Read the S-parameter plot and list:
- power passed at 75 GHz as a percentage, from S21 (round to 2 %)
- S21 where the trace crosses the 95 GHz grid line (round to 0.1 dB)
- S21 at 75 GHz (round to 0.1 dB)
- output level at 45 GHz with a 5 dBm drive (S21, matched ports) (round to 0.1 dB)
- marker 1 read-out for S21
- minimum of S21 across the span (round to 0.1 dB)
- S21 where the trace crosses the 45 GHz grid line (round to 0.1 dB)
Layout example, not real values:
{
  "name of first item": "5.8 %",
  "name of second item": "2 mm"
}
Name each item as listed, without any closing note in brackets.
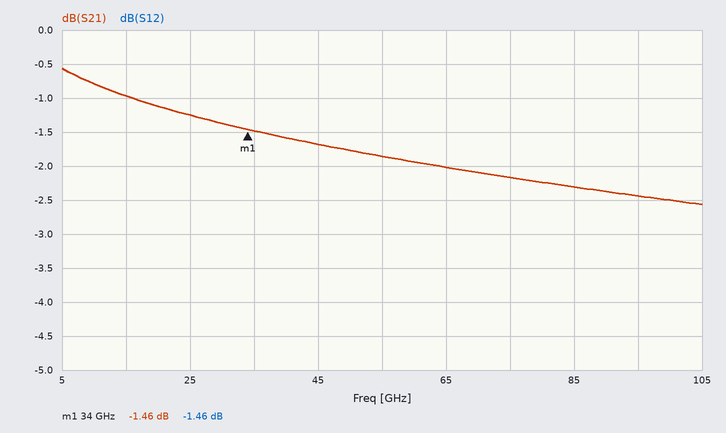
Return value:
{
  "power passed at 75 GHz as a percentage, from S21": "60 %",
  "S21 where the trace crosses the 95 GHz grid line": "-2.4 dB",
  "S21 at 75 GHz": "-2.2 dB",
  "output level at 45 GHz with a 5 dBm drive (S21, matched ports)": "3.3 dBm",
  "marker 1 read-out for S21": "-1.46 dB",
  "minimum of S21 across the span": "-2.6 dB",
  "S21 where the trace crosses the 45 GHz grid line": "-1.7 dB"
}
